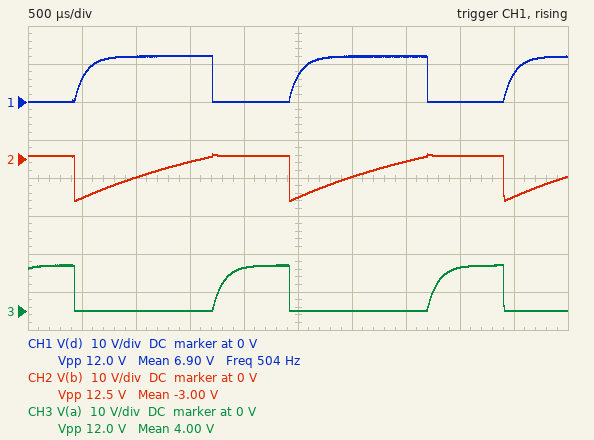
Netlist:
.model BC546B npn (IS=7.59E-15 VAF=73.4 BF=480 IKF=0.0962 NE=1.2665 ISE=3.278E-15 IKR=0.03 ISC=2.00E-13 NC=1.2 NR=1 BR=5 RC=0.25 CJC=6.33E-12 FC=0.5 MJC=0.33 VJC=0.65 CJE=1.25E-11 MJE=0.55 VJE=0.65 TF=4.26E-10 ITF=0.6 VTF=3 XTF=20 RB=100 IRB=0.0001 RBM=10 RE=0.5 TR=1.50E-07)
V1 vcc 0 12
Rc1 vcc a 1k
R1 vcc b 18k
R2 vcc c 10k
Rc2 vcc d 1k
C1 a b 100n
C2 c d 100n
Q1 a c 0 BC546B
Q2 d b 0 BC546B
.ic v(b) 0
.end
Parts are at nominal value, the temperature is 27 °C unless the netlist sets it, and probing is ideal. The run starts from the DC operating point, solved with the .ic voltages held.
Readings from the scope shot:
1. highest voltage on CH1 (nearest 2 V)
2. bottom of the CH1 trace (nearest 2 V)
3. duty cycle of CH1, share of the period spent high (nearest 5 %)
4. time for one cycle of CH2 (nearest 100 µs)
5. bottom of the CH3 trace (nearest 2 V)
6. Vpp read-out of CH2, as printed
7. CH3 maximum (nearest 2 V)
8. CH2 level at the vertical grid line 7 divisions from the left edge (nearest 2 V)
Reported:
12 V
0 V
60 %
2.0 ms
0 V
12.5 V
12 V
0 V
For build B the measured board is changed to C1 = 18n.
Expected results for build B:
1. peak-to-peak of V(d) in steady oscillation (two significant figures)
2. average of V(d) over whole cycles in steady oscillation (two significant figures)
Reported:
11 V
2.0 V
